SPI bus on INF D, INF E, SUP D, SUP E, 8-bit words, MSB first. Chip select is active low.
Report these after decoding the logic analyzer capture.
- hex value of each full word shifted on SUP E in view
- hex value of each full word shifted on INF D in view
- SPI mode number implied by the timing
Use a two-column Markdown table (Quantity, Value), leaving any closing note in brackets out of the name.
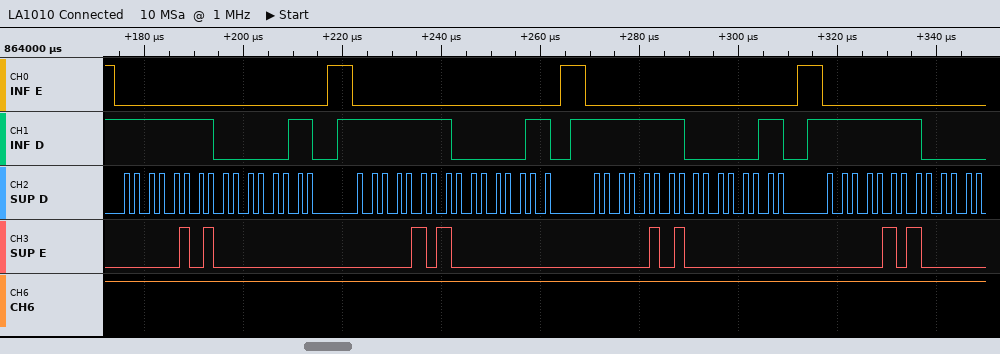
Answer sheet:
| Quantity | Value |
|---|---|
| hex value of each full word shifted on SUP E in view | 05, 00, 05, 00, 05, 00, 05 |
| hex value of each full word shifted on INF D in view | FF, 03, FF, 03, FF, 03, FF |
| SPI mode number implied by the timing | 0 |
